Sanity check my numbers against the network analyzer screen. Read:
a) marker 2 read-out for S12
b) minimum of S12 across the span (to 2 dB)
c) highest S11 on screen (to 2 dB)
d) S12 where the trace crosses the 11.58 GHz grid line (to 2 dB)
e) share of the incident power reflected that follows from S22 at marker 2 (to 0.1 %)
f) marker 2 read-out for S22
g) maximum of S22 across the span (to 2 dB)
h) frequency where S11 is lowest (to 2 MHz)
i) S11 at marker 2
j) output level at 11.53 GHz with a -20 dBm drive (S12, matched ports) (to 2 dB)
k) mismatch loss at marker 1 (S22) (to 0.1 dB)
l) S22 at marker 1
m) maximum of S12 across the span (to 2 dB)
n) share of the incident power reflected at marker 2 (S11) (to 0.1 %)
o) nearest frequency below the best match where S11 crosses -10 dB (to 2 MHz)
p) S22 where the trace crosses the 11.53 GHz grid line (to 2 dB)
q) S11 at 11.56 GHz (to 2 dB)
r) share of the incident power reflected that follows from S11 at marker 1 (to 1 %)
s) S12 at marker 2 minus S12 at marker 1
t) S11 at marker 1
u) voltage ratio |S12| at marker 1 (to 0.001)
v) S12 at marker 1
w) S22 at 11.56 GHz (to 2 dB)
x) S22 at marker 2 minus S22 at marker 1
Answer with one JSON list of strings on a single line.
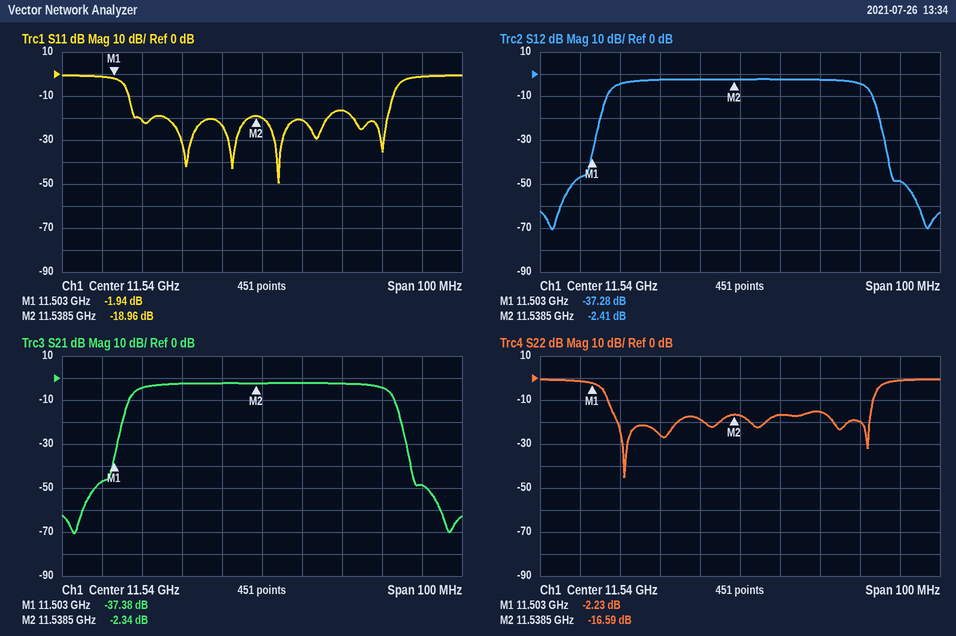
["-2.41 dB", "-70 dB", "0 dB", "-48 dB", "2.2 %", "-16.59 dB", "0 dB", "11.544 GHz", "-18.96 dB", "-22 dBm", "4.0 dB", "-2.23 dB", "-2 dB", "1.3 %", "11.506 GHz", "-18 dB", "-16 dB", "64 %", "34.87 dB", "-1.94 dB", "0.014", "-37.28 dB", "-16 dB", "-14.36 dB"]
